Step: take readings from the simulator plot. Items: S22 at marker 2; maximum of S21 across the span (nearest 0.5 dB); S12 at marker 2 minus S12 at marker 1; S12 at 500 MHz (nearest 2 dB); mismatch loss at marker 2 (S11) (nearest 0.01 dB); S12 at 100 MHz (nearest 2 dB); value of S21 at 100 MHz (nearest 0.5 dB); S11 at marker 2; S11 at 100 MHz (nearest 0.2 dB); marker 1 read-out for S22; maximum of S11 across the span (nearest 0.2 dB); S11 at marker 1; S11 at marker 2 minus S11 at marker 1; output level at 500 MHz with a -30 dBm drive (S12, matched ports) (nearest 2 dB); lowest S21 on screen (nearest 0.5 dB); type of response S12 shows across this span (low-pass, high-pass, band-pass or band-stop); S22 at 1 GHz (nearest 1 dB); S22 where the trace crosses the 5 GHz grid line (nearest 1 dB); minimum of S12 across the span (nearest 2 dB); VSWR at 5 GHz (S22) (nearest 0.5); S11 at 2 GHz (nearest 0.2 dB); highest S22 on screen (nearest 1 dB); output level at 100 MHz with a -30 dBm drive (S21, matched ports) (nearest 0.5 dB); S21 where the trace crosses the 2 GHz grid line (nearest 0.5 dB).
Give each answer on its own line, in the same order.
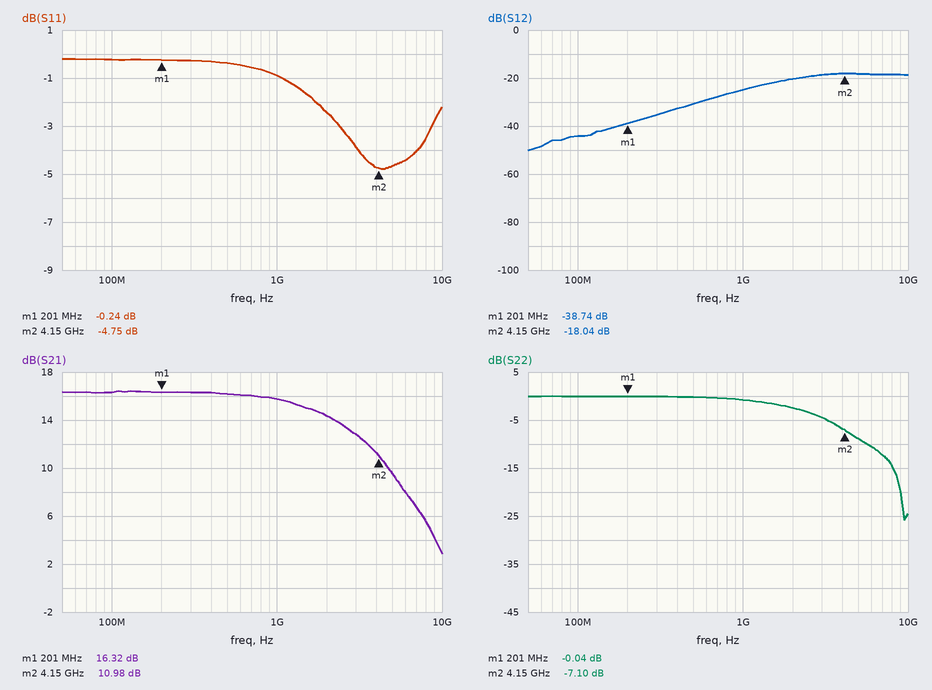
-7.10 dB
16.5 dB
20.70 dB
-30 dB
1.77 dB
-44 dB
16.5 dB
-4.75 dB
-0.2 dB
-0.04 dB
-0.2 dB
-0.24 dB
-4.51 dB
-60 dBm
3.0 dB
high-pass
-1 dB
-9 dB
-50 dB
2.0
-2.4 dB
0 dB
-13.5 dBm
14.5 dB
